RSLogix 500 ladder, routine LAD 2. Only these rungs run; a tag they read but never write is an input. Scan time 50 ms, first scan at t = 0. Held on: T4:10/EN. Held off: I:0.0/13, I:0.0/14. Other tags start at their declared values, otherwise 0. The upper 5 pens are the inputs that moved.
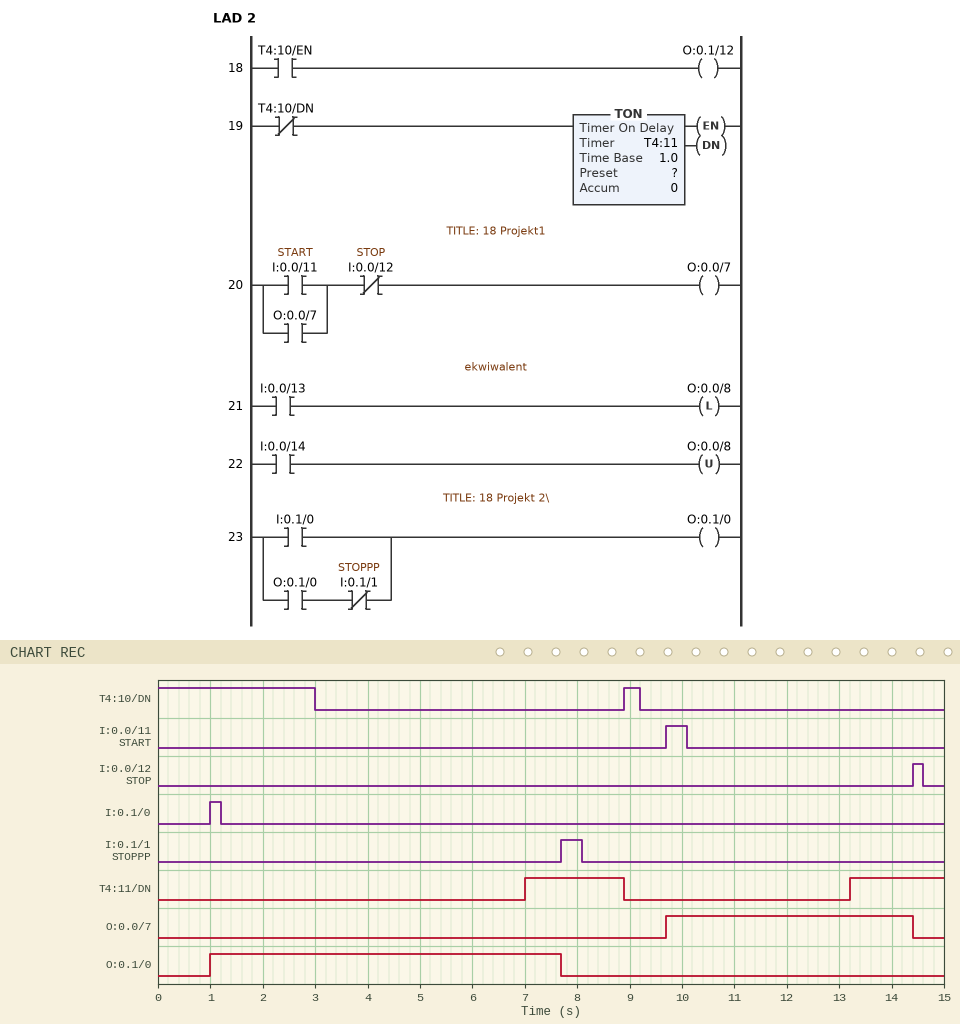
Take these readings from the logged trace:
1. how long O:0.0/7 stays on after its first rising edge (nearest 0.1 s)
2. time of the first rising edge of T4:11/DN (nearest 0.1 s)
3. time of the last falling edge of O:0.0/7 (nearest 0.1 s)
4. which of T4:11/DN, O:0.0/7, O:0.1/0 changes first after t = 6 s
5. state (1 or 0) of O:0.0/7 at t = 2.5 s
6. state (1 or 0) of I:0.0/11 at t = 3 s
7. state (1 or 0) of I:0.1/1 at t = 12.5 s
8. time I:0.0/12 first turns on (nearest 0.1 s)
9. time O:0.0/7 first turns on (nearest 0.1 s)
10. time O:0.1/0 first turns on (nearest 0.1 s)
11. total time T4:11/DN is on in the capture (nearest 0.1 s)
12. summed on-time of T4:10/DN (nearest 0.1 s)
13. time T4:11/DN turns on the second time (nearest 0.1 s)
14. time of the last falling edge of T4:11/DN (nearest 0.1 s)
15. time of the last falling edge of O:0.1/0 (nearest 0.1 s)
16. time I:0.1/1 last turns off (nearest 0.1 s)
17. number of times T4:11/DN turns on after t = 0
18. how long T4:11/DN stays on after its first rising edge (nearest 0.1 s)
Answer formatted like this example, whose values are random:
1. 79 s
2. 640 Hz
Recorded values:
1. 4.7 s
2. 7.0 s
3. 14.4 s
4. T4:11/DN
5. 0
6. 0
7. 0
8. 14.4 s
9. 9.7 s
10. 1.0 s
11. 3.7 s
12. 3.3 s
13. 13.2 s
14. 8.9 s
15. 7.7 s
16. 8.1 s
17. 2
18. 1.9 s
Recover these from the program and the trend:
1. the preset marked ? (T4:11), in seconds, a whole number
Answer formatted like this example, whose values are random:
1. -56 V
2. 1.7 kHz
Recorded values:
1. 4 s
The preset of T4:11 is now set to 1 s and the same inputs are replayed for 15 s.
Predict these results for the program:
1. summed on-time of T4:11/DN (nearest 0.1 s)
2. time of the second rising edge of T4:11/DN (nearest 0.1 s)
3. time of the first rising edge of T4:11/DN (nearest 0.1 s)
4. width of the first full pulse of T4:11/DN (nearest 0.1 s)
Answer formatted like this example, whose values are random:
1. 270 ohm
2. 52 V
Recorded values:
1. 9.7 s
2. 10.2 s
3. 4.0 s
4. 4.9 s
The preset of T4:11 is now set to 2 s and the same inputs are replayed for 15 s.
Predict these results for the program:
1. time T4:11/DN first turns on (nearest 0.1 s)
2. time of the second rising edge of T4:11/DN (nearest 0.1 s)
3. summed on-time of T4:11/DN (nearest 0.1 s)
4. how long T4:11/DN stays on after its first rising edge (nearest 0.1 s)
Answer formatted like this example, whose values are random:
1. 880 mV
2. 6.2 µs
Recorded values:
1. 5.0 s
2. 11.2 s
3. 7.7 s
4. 3.9 s
